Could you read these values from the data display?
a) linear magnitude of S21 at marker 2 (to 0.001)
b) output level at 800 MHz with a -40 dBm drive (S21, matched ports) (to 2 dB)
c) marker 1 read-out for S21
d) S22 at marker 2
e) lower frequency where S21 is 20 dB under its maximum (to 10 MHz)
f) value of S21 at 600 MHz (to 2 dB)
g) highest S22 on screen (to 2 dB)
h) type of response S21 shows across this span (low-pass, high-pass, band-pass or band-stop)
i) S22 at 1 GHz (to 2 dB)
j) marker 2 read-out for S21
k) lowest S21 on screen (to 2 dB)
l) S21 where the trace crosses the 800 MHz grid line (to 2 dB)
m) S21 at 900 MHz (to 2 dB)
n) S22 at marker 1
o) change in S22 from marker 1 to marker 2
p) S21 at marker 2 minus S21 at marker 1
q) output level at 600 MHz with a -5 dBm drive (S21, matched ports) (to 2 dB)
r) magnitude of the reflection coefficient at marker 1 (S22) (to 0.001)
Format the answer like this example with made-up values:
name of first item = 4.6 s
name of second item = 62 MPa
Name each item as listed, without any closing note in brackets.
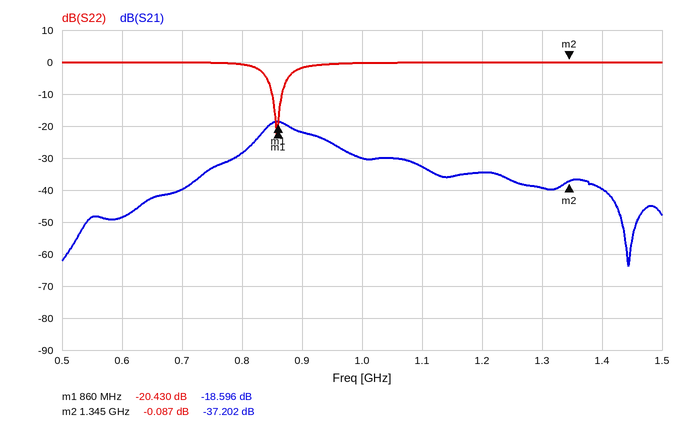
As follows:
linear magnitude of S21 at marker 2 = 0.014
output level at 800 MHz with a -40 dBm drive (S21, matched ports) = -68 dBm
marker 1 read-out for S21 = -18.596 dB
S22 at marker 2 = -0.087 dB
lower frequency where S21 is 20 dB under its maximum = 710 MHz
value of S21 at 600 MHz = -48 dB
highest S22 on screen = 0 dB
type of response S21 shows across this span = band-pass
S22 at 1 GHz = 0 dB
marker 2 read-out for S21 = -37.202 dB
lowest S21 on screen = -64 dB
S21 where the trace crosses the 800 MHz grid line = -28 dB
S21 at 900 MHz = -22 dB
S22 at marker 1 = -20.430 dB
change in S22 from marker 1 to marker 2 = 20.343 dB
S21 at marker 2 minus S21 at marker 1 = -18.606 dB
output level at 600 MHz with a -5 dBm drive (S21, matched ports) = -54 dBm
magnitude of the reflection coefficient at marker 1 (S22) = 0.095
